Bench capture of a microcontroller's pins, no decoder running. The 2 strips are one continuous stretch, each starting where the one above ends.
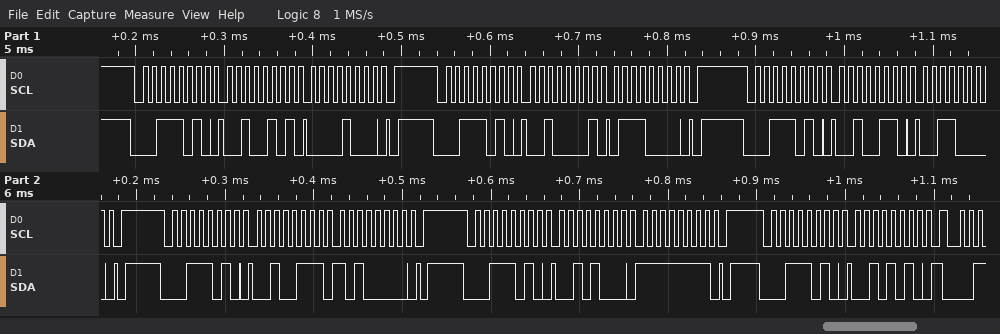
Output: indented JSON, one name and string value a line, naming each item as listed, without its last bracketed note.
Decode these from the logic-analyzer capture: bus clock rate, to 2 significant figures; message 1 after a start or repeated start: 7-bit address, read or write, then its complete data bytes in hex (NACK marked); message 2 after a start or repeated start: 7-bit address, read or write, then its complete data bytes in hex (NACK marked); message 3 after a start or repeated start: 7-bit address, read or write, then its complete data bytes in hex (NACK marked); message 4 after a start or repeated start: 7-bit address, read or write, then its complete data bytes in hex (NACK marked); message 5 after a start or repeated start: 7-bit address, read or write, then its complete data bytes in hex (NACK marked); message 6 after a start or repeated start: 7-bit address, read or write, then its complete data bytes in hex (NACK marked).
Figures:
{
  "bus clock rate, to 2 significant figures": "100 kHz",
  "message 1 after a start or repeated start: 7-bit address, read or write, then its complete data bytes in hex": "0x1D write: 25 08",
  "message 2 after a start or repeated start: 7-bit address, read or write, then its complete data bytes in hex": "0x1D write: 21 70",
  "message 3 after a start or repeated start: 7-bit address, read or write, then its complete data bytes in hex": "0x1D write: 26 30",
  "message 4 after a start or repeated start: 7-bit address, read or write, then its complete data bytes in hex": "0x1D write: 27 A0",
  "message 5 after a start or repeated start: 7-bit address, read or write, then its complete data bytes in hex": "0x1D write: 28 FF",
  "message 6 after a start or repeated start: 7-bit address, read or write, then its complete data bytes in hex": "0x1D write: 2A"
}
